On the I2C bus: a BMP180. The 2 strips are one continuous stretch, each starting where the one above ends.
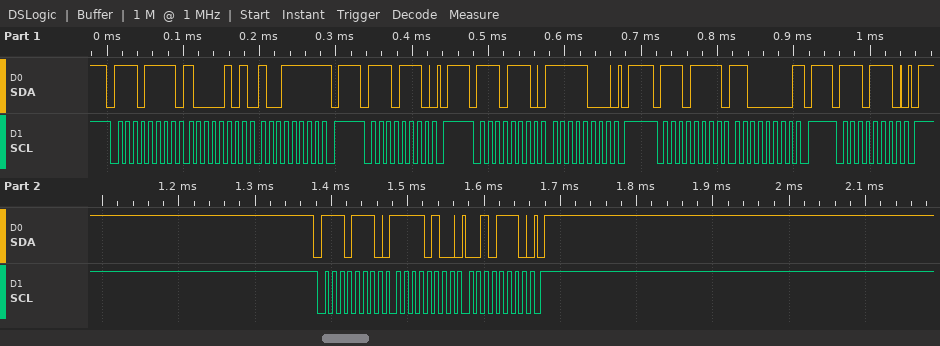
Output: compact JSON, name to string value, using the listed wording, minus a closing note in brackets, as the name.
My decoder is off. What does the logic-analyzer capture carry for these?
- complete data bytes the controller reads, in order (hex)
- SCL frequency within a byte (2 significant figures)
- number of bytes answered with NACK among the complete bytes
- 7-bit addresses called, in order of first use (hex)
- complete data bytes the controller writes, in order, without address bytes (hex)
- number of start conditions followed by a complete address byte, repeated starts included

{"complete data bytes the controller reads, in order": "85 9F C0", "SCL frequency within a byte": "100 kHz", "number of bytes answered with NACK among the complete bytes": "2", "7-bit addresses called, in order of first use": "0x77", "complete data bytes the controller writes, in order, without address bytes": "F8 F4 2E", "number of start conditions followed by a complete address byte, repeated starts included": "6"}
